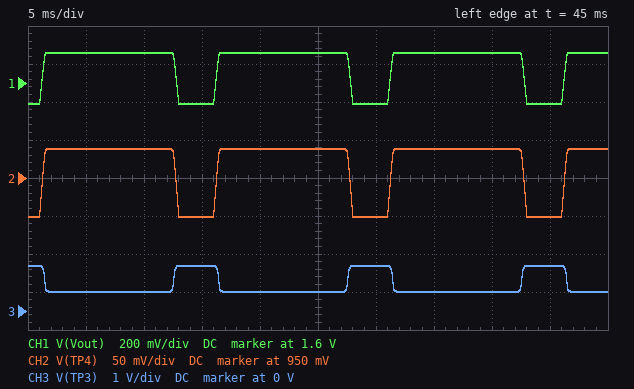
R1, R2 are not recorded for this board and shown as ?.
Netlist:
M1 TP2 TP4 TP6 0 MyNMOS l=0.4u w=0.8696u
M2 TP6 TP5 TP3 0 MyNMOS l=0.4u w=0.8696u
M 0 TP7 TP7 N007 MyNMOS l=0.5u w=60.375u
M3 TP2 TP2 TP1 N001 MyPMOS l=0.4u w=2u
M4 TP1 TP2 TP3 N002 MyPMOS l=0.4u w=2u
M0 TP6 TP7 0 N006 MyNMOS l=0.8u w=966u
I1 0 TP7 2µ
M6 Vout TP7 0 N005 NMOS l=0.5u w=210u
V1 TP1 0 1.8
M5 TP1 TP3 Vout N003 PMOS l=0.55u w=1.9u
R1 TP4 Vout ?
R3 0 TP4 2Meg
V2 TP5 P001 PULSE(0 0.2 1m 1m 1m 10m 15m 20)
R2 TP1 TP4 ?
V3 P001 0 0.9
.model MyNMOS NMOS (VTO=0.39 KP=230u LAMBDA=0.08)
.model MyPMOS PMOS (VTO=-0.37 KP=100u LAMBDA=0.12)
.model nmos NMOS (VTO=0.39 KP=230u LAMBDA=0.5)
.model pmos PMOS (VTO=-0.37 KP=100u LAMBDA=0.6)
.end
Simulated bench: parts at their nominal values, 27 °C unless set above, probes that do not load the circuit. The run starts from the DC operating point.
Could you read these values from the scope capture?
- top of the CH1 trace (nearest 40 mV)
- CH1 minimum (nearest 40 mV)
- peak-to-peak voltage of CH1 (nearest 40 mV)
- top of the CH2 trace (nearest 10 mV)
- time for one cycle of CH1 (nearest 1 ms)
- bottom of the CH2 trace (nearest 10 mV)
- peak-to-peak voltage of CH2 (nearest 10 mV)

1.76 V
1.48 V
280 mV
990 mV
15 ms
900 mV
90 mV
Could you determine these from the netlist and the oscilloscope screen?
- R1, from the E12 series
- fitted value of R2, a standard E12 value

2.7 MΩ
3.9 MΩ
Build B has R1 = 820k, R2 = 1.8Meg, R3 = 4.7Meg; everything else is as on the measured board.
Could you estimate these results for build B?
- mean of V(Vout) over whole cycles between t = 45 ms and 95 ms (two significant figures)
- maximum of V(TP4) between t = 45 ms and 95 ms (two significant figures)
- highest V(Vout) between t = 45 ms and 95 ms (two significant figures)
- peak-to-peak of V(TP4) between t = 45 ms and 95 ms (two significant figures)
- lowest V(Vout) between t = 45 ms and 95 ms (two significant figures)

890 mV
1.1 V
970 mV
200 mV
650 mV
